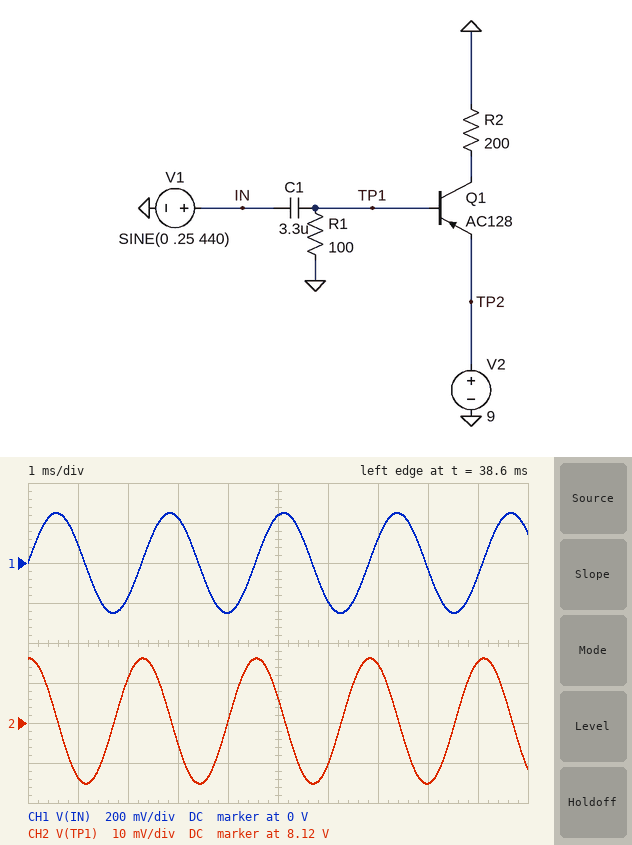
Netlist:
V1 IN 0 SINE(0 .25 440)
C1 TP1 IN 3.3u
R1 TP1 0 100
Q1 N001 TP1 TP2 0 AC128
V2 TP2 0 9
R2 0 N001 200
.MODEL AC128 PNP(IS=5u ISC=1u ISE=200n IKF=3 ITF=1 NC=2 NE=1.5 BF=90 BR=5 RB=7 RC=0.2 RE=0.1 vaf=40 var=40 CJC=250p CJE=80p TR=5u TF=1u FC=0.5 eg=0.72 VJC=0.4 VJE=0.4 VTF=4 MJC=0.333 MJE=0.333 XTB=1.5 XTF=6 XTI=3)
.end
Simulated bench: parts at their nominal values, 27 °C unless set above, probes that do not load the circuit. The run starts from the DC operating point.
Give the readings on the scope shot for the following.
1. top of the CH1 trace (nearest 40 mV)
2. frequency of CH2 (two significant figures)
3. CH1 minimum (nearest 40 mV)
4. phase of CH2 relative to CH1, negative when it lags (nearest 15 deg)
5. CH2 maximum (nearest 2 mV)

240 mV
440 Hz
-240 mV
90 deg
8.136 V
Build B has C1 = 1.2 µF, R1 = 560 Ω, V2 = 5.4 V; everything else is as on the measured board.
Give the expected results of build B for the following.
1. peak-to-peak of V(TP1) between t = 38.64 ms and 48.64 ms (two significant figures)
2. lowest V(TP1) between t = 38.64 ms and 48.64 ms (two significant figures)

15 mV
5.1 V
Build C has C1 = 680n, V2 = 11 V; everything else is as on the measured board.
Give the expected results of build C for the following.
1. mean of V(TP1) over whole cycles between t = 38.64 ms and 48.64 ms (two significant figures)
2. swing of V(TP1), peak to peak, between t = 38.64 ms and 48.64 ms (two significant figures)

10 V
6.4 mV
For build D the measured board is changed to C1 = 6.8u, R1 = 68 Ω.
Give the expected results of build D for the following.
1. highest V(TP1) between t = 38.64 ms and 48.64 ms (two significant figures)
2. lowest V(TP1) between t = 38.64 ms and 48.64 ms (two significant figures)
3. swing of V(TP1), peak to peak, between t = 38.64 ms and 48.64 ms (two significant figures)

7.9 V
7.8 V
62 mV
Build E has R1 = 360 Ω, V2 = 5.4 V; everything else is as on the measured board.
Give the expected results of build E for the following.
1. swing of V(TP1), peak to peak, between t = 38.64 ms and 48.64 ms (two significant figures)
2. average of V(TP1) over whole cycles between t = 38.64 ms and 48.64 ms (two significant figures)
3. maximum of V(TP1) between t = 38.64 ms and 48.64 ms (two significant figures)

38 mV
5.0 V
5.1 V
